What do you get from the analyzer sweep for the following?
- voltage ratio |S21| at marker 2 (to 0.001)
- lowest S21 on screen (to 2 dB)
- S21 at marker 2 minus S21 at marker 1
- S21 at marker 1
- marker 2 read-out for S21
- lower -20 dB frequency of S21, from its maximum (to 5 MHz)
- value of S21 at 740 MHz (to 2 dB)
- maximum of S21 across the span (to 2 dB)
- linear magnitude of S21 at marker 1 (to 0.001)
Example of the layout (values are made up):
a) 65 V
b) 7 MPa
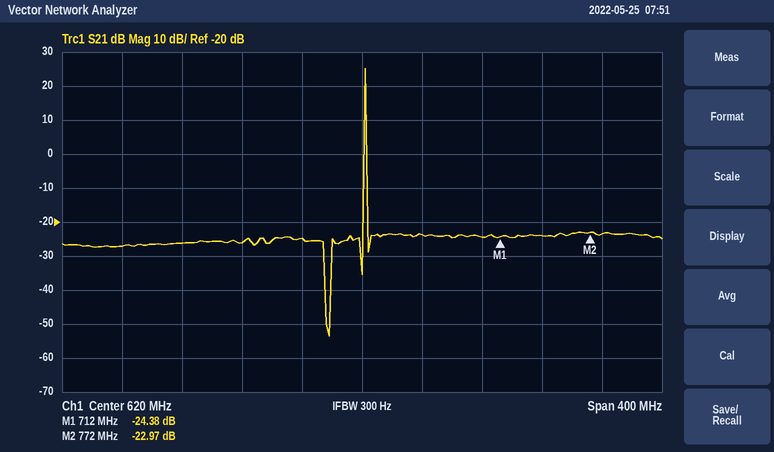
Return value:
a) 0.071
b) -54 dB
c) 1.41 dB
d) -24.38 dB
e) -22.97 dB
f) 620 MHz
g) -24 dB
h) 26 dB
i) 0.060
